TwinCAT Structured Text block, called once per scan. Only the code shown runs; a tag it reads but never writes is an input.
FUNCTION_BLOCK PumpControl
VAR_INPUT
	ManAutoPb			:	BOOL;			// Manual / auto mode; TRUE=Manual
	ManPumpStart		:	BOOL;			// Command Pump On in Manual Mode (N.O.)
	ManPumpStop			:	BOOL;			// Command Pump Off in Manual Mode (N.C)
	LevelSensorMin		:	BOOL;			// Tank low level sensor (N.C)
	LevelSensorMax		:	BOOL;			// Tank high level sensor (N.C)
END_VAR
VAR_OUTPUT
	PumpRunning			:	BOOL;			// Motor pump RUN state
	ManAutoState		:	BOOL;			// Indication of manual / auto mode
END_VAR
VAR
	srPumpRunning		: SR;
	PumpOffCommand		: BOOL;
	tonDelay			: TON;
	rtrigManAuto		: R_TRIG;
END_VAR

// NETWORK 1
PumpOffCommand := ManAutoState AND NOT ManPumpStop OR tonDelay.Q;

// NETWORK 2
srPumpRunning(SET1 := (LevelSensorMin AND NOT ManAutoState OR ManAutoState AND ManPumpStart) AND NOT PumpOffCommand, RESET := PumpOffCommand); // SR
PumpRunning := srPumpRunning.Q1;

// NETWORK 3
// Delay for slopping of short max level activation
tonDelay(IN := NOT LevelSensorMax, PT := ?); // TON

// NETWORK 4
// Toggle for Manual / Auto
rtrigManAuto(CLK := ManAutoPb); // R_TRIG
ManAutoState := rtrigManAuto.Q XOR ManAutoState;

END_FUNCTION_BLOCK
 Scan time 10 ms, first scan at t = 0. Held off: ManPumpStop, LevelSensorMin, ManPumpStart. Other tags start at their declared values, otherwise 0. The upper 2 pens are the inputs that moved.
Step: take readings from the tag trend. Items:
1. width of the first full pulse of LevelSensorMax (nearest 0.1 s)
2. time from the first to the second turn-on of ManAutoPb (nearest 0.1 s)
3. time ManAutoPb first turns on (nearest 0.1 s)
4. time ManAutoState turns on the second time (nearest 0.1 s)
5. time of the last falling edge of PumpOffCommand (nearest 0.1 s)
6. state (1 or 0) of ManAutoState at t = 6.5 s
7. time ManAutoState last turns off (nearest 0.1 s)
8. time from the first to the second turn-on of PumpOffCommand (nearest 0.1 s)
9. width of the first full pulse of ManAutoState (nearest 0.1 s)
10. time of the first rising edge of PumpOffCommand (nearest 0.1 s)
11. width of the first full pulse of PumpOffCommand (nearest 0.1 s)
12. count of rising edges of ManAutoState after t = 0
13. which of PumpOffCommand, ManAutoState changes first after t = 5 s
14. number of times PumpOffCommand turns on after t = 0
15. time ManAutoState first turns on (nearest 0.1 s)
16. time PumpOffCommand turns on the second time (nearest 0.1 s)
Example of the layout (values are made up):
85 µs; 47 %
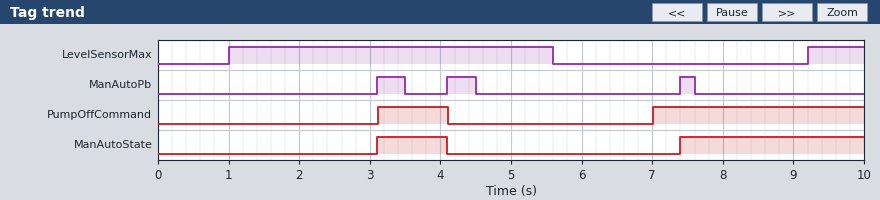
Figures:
4.6 s; 1.0 s; 3.1 s; 7.4 s; 4.1 s; 0; 4.1 s; 3.9 s; 1.0 s; 3.1 s; 1.0 s; 2; PumpOffCommand; 2; 3.1 s; 7.0 s
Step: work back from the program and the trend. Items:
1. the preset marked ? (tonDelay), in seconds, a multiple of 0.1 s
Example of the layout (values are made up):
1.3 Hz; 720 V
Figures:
1.4 s
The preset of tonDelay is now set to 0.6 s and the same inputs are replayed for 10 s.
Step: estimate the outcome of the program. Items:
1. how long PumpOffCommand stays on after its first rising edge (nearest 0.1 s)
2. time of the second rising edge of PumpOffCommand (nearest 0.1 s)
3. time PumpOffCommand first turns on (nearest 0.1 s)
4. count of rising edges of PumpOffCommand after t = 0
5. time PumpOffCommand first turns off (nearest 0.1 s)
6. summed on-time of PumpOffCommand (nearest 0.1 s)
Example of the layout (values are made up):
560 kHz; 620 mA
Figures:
0.4 s; 3.1 s; 0.6 s; 3; 1.0 s; 5.2 s
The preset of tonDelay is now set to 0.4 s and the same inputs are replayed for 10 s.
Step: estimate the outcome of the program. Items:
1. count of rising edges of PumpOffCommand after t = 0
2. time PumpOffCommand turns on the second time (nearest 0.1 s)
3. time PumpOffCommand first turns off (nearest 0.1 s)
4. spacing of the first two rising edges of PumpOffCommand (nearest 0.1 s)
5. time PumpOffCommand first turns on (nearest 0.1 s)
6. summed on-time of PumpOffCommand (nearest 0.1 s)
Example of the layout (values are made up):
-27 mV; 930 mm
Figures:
3; 3.1 s; 1.0 s; 2.7 s; 0.4 s; 5.6 s
